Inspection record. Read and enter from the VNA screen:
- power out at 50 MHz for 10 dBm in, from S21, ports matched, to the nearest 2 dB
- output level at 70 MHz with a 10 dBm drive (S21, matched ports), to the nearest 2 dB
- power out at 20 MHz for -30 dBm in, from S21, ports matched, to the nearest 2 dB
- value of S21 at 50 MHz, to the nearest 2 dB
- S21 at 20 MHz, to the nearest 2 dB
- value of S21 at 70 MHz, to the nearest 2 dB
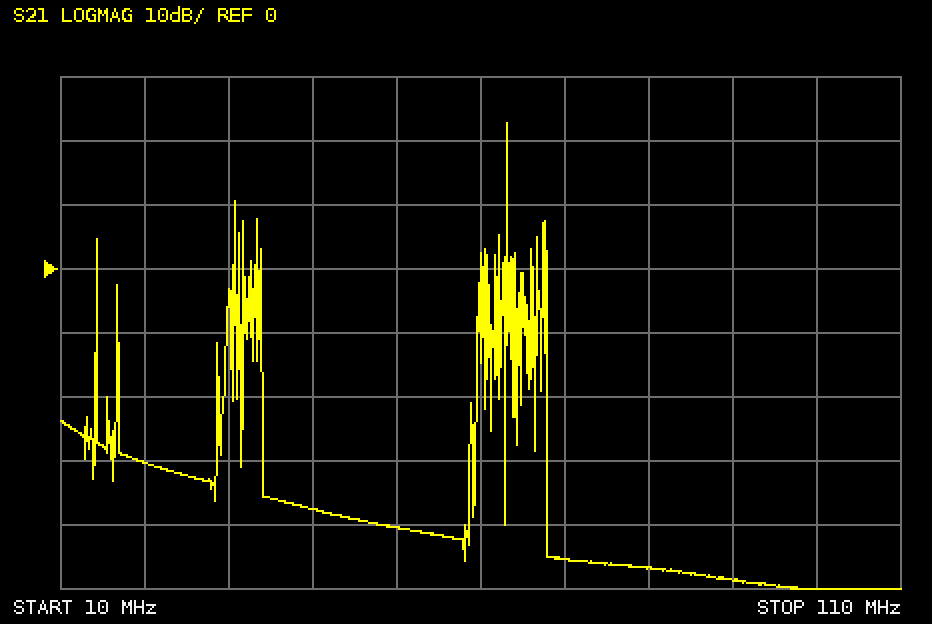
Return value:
-30 dBm
-36 dBm
-60 dBm
-40 dB
-30 dB
-46 dB
